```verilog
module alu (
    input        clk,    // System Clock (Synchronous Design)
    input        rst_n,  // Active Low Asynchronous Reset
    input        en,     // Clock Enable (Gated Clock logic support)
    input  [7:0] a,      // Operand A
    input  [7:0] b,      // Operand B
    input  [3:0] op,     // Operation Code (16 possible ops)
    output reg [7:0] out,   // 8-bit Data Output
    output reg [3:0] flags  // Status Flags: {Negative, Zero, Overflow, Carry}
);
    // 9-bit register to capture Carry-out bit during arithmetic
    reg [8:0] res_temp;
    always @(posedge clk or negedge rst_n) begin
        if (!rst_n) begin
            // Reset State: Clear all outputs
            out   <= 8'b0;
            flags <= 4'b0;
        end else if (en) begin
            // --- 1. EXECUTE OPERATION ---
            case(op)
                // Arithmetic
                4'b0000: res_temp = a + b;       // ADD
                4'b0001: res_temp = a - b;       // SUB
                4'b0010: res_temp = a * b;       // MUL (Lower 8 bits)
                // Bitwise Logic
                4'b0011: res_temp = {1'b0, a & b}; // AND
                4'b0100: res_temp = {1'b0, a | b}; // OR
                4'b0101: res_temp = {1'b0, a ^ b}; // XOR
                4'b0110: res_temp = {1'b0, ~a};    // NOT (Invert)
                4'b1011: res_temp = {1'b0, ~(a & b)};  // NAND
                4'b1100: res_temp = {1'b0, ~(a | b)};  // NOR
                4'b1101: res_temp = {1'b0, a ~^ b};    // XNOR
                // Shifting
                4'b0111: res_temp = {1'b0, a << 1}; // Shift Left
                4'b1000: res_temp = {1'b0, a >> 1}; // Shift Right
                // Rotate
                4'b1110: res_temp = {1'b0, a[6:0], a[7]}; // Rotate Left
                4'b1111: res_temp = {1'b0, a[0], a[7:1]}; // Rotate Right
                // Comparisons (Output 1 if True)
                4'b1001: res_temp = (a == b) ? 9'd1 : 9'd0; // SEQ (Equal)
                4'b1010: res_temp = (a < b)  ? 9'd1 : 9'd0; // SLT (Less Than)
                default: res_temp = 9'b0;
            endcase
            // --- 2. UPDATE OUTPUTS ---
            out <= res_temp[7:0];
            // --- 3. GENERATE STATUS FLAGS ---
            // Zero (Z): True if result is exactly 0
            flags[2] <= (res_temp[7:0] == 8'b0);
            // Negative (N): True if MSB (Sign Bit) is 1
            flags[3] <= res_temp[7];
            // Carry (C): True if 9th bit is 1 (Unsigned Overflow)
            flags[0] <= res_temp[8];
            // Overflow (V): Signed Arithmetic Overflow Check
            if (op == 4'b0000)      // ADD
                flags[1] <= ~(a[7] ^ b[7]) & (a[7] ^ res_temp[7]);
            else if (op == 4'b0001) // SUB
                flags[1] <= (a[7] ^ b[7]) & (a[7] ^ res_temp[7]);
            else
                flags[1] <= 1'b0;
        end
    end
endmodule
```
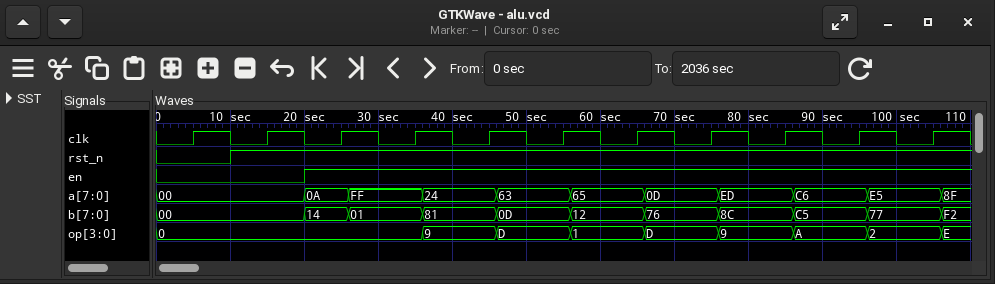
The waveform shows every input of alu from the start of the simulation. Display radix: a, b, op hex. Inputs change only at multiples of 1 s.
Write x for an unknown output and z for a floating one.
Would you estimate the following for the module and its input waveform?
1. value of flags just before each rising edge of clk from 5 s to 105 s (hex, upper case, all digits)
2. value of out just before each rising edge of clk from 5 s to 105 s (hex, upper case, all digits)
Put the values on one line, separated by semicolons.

0, 0, 0, 0, 5, 4, 8, 0, 8, 4, 4; 00, 00, 00, 1E, 00, 00, 91, 53, 84, 00, 00
